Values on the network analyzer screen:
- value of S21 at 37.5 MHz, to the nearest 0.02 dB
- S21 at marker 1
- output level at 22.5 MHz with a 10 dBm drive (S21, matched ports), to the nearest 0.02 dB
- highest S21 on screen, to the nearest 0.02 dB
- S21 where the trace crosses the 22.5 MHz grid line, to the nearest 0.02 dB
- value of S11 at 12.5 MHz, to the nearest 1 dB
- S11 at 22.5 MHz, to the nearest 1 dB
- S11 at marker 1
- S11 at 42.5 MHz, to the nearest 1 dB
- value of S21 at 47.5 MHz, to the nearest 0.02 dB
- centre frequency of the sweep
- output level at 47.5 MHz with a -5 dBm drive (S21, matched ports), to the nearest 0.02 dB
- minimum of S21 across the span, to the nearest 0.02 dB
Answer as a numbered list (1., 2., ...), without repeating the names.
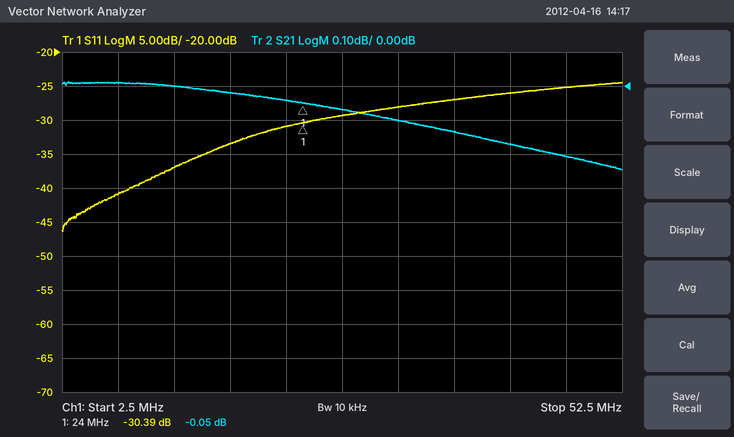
1. -0.14 dB
2. -0.05 dB
3. 9.96 dBm
4. 0.02 dB
5. -0.04 dB
6. -37 dB
7. -31 dB
8. -30.39 dB
9. -26 dB
10. -0.20 dB
11. 27.5 MHz
12. -5.20 dBm
13. -0.24 dB
